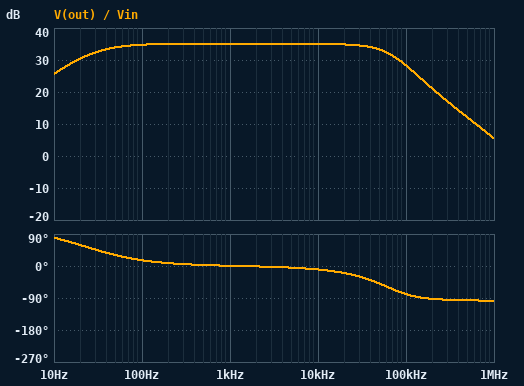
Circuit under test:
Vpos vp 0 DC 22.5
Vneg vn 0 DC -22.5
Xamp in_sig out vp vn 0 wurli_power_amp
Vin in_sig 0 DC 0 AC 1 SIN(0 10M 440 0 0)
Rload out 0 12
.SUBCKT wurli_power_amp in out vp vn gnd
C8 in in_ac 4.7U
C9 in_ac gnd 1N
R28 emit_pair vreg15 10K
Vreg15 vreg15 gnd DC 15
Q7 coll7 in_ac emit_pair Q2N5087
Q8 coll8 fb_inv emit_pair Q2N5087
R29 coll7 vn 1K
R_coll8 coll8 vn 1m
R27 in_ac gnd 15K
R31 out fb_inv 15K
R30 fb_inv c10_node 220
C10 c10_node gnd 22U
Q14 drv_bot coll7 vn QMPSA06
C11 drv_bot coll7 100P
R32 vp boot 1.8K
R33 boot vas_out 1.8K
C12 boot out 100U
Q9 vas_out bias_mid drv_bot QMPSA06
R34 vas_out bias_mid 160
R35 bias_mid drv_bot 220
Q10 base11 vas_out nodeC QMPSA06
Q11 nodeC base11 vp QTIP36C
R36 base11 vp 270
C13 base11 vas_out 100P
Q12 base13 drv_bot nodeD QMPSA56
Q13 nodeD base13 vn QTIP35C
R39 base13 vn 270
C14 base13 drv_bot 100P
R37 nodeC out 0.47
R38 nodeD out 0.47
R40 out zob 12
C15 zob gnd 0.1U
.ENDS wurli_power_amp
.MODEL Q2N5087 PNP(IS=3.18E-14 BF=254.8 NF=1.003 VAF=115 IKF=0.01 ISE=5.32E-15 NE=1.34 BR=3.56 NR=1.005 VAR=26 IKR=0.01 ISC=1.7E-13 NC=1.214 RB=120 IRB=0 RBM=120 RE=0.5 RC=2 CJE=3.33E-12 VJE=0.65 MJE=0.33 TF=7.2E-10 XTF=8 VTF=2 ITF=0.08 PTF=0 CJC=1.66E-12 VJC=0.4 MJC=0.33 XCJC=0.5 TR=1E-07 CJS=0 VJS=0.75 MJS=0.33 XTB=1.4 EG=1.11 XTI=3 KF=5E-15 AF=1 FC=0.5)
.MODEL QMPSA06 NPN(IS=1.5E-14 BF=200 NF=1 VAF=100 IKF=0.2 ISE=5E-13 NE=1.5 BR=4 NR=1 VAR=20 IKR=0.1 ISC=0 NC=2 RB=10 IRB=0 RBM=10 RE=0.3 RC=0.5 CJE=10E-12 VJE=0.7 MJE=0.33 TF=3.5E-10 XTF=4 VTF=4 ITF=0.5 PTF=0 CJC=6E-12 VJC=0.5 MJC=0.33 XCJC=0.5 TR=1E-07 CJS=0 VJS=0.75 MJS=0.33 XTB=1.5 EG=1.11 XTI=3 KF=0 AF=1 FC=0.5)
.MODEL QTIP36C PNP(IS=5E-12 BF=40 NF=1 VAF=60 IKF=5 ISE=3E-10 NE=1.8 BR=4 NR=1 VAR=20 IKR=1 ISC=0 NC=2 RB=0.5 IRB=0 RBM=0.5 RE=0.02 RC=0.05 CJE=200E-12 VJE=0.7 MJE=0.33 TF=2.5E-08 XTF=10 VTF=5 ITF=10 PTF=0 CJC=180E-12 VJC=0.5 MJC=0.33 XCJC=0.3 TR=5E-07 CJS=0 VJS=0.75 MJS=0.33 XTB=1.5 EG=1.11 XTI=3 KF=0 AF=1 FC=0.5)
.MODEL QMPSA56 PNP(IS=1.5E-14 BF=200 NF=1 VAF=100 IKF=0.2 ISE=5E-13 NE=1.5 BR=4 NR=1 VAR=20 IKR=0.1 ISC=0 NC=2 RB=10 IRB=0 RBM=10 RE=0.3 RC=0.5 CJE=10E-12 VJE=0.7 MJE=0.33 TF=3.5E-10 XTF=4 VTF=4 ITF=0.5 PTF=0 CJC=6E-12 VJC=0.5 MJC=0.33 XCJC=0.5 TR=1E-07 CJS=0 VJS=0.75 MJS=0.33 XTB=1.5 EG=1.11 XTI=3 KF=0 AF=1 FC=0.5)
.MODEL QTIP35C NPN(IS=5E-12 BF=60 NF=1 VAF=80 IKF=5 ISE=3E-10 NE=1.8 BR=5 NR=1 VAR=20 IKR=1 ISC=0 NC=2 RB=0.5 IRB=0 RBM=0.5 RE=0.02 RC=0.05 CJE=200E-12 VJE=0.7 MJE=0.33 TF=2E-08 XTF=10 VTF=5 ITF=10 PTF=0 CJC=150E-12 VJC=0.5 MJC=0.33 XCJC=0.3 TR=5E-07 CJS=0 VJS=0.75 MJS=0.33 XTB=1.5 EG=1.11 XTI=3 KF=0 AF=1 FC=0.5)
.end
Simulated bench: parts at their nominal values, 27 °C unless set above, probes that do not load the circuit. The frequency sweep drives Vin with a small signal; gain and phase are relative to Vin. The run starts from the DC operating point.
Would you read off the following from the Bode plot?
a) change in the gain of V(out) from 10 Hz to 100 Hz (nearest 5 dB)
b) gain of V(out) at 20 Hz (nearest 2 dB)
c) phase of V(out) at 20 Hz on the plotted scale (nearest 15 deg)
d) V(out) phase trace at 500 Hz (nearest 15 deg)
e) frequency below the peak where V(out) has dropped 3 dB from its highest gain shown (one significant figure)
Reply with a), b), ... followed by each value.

a) 10 dB
b) 30 dB
c) 60 deg
d) 0 deg
e) 30 Hz
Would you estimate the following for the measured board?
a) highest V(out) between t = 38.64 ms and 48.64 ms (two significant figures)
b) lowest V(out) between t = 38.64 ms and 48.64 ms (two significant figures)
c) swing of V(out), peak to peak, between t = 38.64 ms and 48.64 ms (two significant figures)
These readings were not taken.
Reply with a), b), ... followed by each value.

a) 690 mV
b) -680 mV
c) 1.4 V
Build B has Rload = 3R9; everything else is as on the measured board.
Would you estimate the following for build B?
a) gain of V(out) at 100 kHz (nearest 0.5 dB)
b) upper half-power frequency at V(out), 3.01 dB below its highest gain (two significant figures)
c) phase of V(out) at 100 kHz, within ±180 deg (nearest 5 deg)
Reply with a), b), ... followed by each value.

a) 29.0 dB
b) 65 kHz
c) -65 deg
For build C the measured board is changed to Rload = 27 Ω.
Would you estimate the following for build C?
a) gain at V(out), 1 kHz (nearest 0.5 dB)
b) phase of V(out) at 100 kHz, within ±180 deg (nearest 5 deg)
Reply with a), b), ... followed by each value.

a) 35.5 dB
b) -90 deg
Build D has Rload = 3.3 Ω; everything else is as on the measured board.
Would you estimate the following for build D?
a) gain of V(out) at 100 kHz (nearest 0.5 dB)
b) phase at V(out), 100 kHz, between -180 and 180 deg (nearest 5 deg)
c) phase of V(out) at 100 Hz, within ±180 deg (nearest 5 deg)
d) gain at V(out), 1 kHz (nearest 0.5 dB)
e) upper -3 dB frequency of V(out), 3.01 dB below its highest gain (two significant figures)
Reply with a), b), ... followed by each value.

a) 32.0 dB
b) -55 deg
c) 15 deg
d) 35.5 dB
e) 88 kHz
